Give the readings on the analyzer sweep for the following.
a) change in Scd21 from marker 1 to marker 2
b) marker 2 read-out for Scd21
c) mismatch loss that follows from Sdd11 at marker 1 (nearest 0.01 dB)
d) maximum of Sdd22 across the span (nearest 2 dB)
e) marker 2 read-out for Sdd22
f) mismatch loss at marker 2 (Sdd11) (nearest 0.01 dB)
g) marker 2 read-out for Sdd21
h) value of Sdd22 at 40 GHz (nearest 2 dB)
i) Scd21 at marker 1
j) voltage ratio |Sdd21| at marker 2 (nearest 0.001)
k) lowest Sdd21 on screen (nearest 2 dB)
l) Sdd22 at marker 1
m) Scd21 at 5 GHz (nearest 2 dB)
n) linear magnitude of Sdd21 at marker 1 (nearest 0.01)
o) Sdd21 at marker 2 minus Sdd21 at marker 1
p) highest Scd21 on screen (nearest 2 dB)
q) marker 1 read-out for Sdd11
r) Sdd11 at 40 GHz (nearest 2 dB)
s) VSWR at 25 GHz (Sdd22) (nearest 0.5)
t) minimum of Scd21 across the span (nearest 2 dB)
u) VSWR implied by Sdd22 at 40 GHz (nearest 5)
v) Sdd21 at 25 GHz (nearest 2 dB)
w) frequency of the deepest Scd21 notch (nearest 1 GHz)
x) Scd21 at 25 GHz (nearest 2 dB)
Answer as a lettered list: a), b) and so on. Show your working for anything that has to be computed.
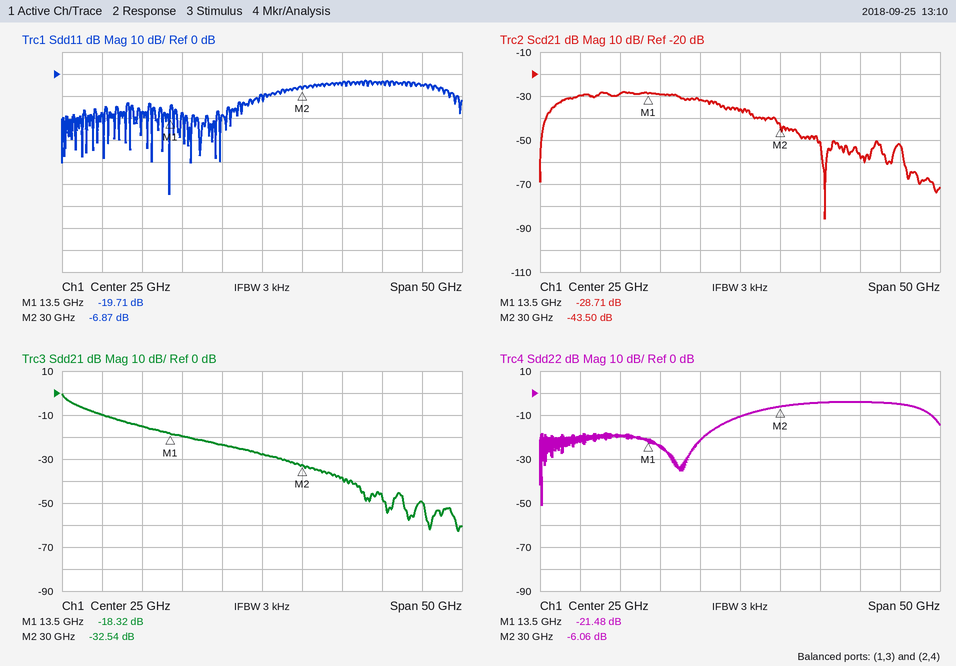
a) -43.5 − (-28.71) = -14.79 dB
b) -43.50 dB
c) −10 log10(1 − 10^(-19.71/10)) ≈ 0.05 dB
d) -4 dB
e) -6.06 dB
f) −10 log10(1 − 10^(-6.87/10)) ≈ 1.00 dB
g) -32.54 dB
h) -4 dB
i) -28.71 dB
j) 10^(-32.54/20) ≈ 0.024
k) -62 dB
l) -21.48 dB
m) -30 dB
n) 10^(-18.32/20) ≈ 0.12
o) -32.54 − (-18.32) = -14.22 dB
p) -28 dB
q) -19.71 dB
r) -4 dB
s) |Γ| = 10^(-10/20) = 0.3162; VSWR = (1 + 0.3162)/(1 − 0.3162) ≈ 1.92, so 2.0 to the nearest 0.5
t) -86 dB
u) |Γ| = 10^(-4/20) = 0.6310; VSWR = (1 + 0.6310)/(1 − 0.6310) ≈ 4.42, so 5 to the nearest 5
v) -28 dB
w) 36 GHz
x) -36 dB
